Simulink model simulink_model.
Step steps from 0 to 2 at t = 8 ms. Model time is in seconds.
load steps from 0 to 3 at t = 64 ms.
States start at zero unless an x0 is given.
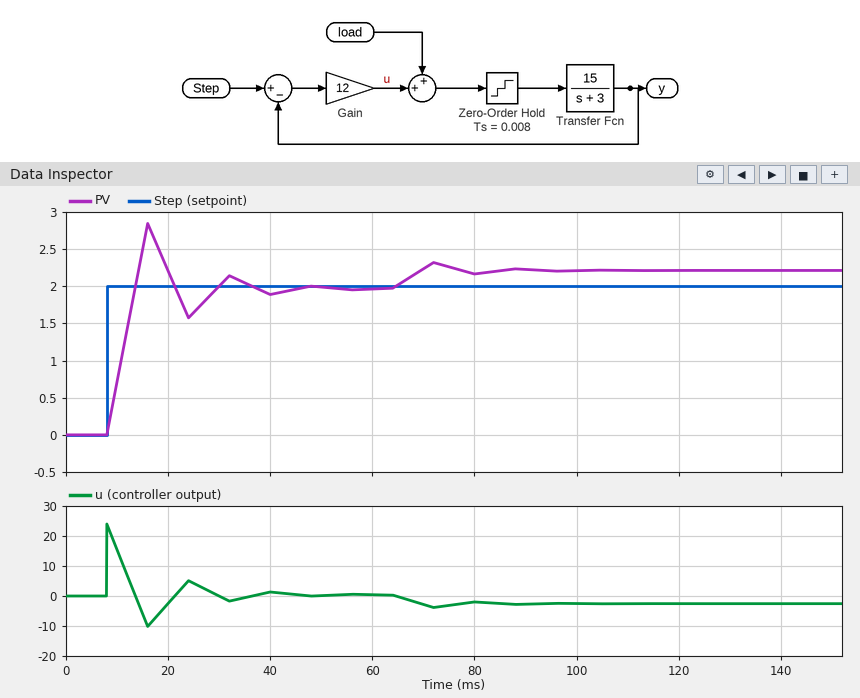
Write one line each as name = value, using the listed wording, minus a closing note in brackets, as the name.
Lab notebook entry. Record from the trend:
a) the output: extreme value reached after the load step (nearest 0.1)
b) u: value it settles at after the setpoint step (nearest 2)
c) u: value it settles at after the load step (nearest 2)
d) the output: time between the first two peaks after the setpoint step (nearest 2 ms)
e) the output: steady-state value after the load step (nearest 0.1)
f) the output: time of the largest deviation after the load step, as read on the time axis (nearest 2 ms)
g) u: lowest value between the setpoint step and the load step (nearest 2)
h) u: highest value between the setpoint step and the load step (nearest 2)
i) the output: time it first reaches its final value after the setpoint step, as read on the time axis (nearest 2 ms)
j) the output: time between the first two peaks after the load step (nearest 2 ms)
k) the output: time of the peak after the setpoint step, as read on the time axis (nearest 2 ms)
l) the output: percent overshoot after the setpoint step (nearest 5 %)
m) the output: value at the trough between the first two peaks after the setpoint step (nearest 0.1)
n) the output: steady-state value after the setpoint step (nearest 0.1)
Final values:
the output: extreme value reached after the load step = 2.3
u: value it settles at after the setpoint step = 0
u: value it settles at after the load step = -2
the output: time between the first two peaks after the setpoint step = 16 ms
the output: steady-state value after the load step = 2.2
the output: time of the largest deviation after the load step, as read on the time axis = 72 ms
u: lowest value between the setpoint step and the load step = -10
u: highest value between the setpoint step and the load step = 24
the output: time it first reaches its final value after the setpoint step, as read on the time axis = 14 ms
the output: time between the first two peaks after the load step = 16 ms
the output: time of the peak after the setpoint step, as read on the time axis = 16 ms
the output: percent overshoot after the setpoint step = 45 %
the output: value at the trough between the first two peaks after the setpoint step = 1.6
the output: steady-state value after the setpoint step = 2.0
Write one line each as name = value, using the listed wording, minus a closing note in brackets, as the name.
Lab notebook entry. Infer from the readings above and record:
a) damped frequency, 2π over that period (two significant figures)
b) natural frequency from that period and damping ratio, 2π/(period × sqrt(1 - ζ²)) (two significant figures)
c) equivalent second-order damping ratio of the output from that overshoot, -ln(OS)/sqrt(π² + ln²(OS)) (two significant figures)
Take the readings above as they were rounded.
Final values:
damped frequency, 2π over that period = 0.39 rad/ms
natural frequency from that period and damping ratio, 2π/(period × sqrt(1 - ζ²)) = 0.41 rad/ms
equivalent second-order damping ratio of the output from that overshoot, -ln(OS)/sqrt(π² + ln²(OS)) = 0.25
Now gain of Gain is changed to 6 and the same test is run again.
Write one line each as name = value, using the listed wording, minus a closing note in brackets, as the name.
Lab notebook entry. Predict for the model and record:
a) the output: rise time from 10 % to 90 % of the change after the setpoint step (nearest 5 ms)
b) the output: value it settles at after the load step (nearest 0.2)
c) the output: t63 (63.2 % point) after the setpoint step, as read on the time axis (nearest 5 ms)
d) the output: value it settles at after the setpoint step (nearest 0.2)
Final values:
the output: rise time from 10 % to 90 % of the change after the setpoint step = 15 ms
the output: value it settles at after the load step = 2.4
the output: t63 (63.2 % point) after the setpoint step, as read on the time axis = 15 ms
the output: value it settles at after the setpoint step = 2.0
